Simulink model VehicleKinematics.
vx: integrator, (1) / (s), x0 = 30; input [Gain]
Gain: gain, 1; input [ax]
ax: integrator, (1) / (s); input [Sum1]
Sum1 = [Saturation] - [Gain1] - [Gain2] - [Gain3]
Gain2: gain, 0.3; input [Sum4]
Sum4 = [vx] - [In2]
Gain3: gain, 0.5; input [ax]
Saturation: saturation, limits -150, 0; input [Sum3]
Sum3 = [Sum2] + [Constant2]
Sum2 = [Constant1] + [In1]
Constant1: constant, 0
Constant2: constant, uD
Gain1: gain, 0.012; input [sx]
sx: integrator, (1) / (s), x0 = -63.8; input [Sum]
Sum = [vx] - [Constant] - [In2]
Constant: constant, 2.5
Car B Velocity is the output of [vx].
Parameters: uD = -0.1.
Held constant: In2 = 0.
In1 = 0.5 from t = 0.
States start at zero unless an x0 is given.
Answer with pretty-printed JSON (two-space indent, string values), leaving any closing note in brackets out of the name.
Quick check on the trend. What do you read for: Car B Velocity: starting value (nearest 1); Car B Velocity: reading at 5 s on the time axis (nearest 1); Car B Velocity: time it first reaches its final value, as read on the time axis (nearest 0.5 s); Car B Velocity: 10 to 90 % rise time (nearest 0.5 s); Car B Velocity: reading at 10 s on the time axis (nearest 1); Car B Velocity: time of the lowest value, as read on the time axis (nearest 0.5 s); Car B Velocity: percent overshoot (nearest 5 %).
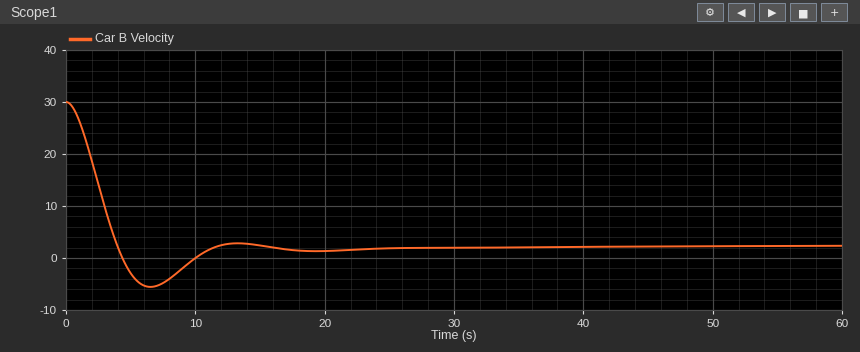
{
  "Car B Velocity: starting value": "30",
  "Car B Velocity: reading at 5 s on the time axis": "-3",
  "Car B Velocity: time it first reaches its final value, as read on the time axis": "4.0 s",
  "Car B Velocity: 10 to 90 % rise time": "2.5 s",
  "Car B Velocity: reading at 10 s on the time axis": "0",
  "Car B Velocity: time of the lowest value, as read on the time axis": "6.5 s",
  "Car B Velocity: percent overshoot": "30 %"
}
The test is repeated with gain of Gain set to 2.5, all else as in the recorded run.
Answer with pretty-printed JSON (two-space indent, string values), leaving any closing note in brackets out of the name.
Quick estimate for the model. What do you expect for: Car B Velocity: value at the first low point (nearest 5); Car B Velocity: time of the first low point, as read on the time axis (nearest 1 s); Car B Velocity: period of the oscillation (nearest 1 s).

{
  "Car B Velocity: value at the first low point": "-10",
  "Car B Velocity: time of the first low point, as read on the time axis": "4 s",
  "Car B Velocity: period of the oscillation": "8 s"
}
